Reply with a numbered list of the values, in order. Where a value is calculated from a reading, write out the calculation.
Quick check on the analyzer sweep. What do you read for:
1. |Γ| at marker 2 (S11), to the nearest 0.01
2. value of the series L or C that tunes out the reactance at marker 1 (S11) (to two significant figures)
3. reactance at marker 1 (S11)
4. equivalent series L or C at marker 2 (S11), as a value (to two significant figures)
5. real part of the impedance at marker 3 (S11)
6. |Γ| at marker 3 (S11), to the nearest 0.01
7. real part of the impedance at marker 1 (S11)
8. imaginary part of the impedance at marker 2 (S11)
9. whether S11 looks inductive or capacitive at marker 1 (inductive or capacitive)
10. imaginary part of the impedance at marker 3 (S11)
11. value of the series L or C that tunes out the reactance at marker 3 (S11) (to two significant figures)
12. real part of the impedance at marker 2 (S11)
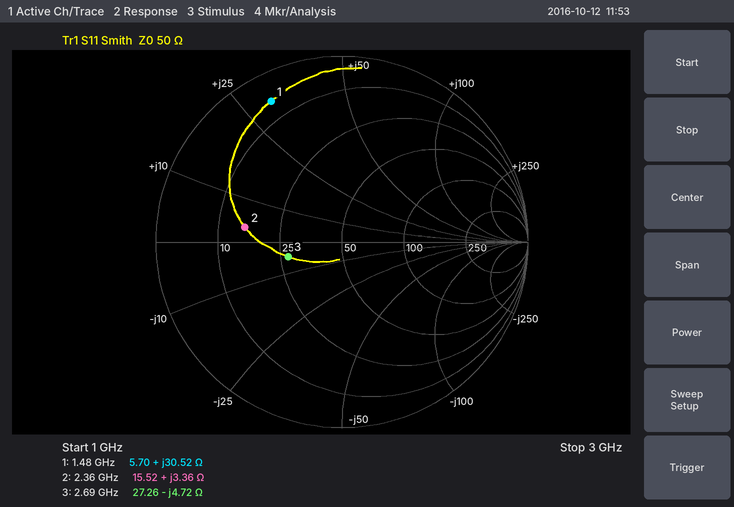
1. 0.53
2. C = 1/(2π × 1.48 GHz × 30.52 Ω) ≈ 3.5 pF
3. +30.52 Ω
4. L = 3.36 Ω/(2π × 2.36 GHz) ≈ 227 pH, so 230 pH to two significant figures
5. 27.26 Ω
6. 0.30
7. 5.70 Ω
8. +3.36 Ω
9. inductive
10. -4.72 Ω
11. L = 4.72 Ω/(2π × 2.69 GHz) ≈ 279 pH, so 280 pH to two significant figures
12. 15.52 Ω
